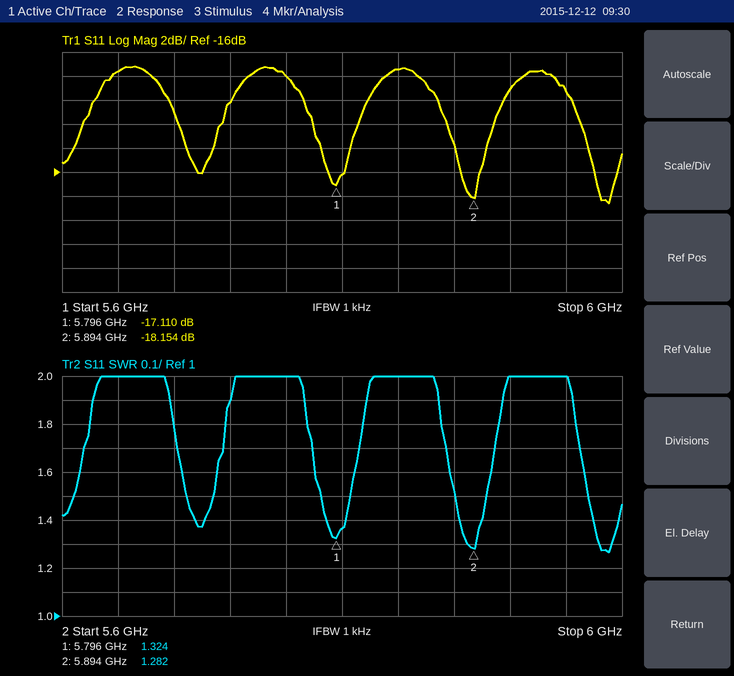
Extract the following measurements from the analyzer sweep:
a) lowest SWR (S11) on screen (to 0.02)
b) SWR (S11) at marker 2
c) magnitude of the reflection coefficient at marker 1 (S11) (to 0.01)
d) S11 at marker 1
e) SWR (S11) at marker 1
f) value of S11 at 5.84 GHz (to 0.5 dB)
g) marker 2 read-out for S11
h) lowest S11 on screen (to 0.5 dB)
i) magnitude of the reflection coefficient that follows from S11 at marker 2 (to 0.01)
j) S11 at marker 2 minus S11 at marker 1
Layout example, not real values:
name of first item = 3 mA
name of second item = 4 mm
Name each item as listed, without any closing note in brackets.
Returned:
lowest SWR (S11) on screen = 1.26
SWR (S11) at marker 2 = 1.282
magnitude of the reflection coefficient at marker 1 (S11) = 0.14
S11 at marker 1 = -17.110 dB
SWR (S11) at marker 1 = 1.324
value of S11 at 5.84 GHz = -7.5 dB
marker 2 read-out for S11 = -18.154 dB
lowest S11 on screen = -18.5 dB
magnitude of the reflection coefficient that follows from S11 at marker 2 = 0.12
S11 at marker 2 minus S11 at marker 1 = -1.044 dB
